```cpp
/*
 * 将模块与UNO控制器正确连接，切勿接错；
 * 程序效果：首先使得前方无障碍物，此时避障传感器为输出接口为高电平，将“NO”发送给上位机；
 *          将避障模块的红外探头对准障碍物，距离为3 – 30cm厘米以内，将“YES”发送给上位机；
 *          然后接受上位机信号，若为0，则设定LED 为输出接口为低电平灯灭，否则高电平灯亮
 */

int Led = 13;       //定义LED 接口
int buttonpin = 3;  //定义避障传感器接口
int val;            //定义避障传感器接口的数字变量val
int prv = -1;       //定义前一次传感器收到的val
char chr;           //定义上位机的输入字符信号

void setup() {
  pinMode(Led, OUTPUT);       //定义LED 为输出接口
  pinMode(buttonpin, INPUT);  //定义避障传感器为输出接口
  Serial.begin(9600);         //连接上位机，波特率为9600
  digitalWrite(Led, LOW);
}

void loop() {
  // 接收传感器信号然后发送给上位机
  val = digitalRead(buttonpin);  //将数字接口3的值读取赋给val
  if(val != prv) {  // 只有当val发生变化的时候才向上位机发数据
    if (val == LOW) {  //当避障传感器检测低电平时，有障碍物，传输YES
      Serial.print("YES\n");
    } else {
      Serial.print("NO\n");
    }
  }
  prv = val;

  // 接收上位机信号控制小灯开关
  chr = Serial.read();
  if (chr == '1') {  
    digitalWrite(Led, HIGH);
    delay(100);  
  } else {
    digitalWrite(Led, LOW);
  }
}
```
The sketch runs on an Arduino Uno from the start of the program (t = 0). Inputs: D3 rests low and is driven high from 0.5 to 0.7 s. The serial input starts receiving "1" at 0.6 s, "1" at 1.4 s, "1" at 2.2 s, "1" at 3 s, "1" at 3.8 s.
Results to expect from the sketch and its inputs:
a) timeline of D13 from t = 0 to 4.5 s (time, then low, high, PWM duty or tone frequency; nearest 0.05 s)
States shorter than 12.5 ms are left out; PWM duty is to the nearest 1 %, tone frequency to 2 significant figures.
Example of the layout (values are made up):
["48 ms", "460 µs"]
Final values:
["0 s low; 0.6 s high; 0.7 s low; 1.4 s high; 1.5 s low; 2.2 s high; 2.3 s low; 3 s high; 3.1 s low; 3.8 s high; 3.9 s low"]
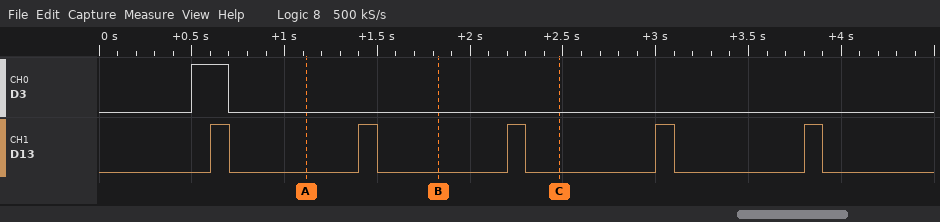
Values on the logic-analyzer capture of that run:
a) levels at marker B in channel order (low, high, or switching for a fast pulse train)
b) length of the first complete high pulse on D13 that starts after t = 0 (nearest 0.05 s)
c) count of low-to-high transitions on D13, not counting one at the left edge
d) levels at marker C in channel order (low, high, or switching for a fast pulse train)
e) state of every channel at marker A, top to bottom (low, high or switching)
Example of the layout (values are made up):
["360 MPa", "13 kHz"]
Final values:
["D3 low, D13 low", "0.10 s", "5", "D3 low, D13 low", "D3 low, D13 low"]
